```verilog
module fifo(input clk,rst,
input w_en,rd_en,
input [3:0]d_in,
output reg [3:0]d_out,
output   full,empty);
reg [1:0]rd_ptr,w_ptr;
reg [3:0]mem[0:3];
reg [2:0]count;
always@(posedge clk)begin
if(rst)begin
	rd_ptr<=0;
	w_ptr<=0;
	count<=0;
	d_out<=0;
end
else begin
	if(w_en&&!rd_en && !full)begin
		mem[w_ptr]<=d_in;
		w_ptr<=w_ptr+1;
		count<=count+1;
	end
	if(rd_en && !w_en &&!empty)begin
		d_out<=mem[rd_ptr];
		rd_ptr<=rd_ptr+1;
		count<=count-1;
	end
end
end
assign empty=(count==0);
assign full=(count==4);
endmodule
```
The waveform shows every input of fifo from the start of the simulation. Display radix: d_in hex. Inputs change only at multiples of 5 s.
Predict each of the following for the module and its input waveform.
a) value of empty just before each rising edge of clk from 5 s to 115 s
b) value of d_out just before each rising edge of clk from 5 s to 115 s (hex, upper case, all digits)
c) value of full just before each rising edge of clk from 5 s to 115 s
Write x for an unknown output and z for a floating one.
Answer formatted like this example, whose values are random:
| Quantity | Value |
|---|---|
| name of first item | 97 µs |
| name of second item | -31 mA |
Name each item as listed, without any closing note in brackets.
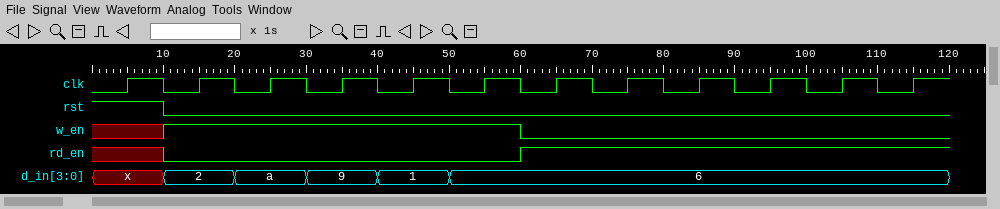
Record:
| Quantity | Value |
|---|---|
| value of empty just before each rising edge of clk from 5 s to 115 s | x 1 0 0 0 0 0 0 0 0 1 1 |
| value of d_out just before each rising edge of clk from 5 s to 115 s | x, 0, 0, 0, 0, 0, 0, 2, A, 9, 1, 1 |
| value of full just before each rising edge of clk from 5 s to 115 s | x 0 0 0 0 1 1 0 0 0 0 0 |
